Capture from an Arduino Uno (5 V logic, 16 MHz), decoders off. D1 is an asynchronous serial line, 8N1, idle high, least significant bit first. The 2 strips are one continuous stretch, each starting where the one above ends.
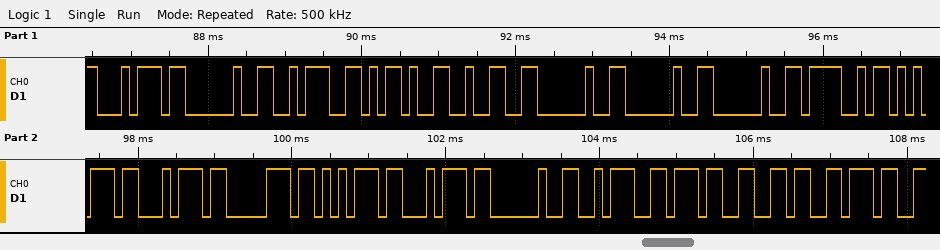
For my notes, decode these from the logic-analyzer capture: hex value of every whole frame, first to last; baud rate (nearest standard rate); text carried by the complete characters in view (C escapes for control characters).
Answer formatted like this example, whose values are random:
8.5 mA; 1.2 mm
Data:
74 20 3A 2D 32 20 20 20 4F 75 74 70 75 74 20 3A 37 36 37; 9600 baud; "t :-2   Output :767"
